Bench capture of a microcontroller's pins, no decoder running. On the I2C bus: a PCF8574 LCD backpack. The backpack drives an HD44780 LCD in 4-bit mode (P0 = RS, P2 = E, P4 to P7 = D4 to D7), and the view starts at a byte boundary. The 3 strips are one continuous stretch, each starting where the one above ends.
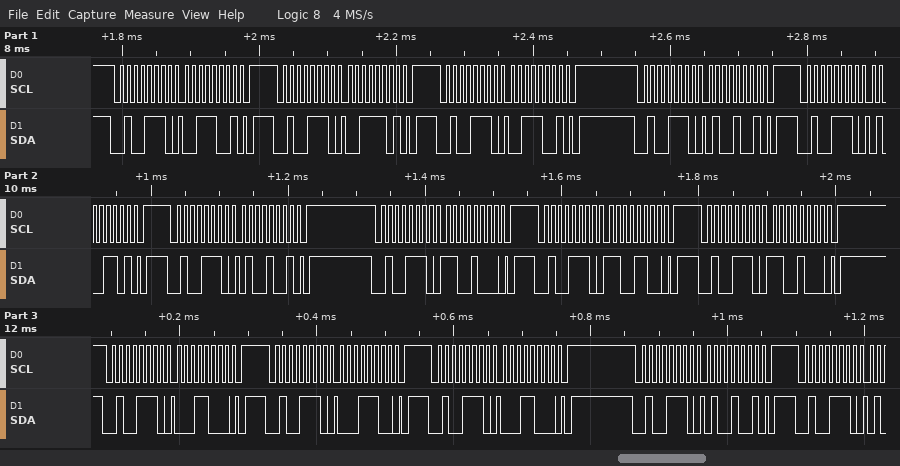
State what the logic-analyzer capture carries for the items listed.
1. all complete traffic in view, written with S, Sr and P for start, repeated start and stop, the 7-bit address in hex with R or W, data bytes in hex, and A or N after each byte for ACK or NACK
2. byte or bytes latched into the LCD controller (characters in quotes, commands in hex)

S 27W A 39 A P S 27W A 3D A P S 27W A 39 A P S 27W A 49 A P S 27W A 4D A P S 27W A 49 A P S 27W A C8 A P S 27W A CC A P S 27W A C8 A P S 27W A 18 A P S 27W A 1C A P S 27W A 18 A P S 27W A 49 A P S 27W A
'4' 0xC1
